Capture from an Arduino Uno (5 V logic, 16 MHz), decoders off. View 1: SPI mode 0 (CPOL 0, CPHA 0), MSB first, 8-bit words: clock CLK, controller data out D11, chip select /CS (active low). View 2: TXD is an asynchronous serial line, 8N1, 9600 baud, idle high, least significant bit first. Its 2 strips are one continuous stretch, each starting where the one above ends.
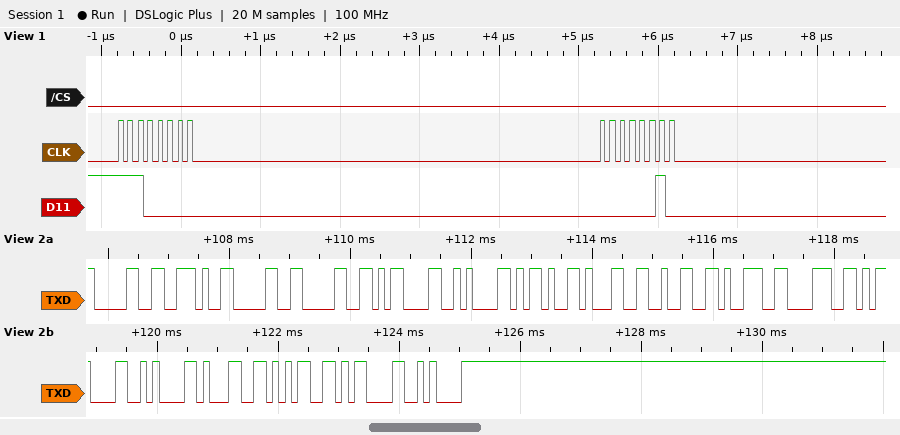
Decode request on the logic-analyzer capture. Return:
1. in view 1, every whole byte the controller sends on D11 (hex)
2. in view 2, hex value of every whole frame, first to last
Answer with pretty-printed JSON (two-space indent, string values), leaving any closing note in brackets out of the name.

{
  "in view 1, every whole byte the controller sends on D11": "E0 02",
  "in view 2, hex value of every whole frame, first to last": "0x30 0x2E 0x30 0x30 0x0D 0x0A 0x2D 0x31 0x32 0x39 0x38 0x0D 0x0A 0x31 0x35 0x0D 0x0A"
}
